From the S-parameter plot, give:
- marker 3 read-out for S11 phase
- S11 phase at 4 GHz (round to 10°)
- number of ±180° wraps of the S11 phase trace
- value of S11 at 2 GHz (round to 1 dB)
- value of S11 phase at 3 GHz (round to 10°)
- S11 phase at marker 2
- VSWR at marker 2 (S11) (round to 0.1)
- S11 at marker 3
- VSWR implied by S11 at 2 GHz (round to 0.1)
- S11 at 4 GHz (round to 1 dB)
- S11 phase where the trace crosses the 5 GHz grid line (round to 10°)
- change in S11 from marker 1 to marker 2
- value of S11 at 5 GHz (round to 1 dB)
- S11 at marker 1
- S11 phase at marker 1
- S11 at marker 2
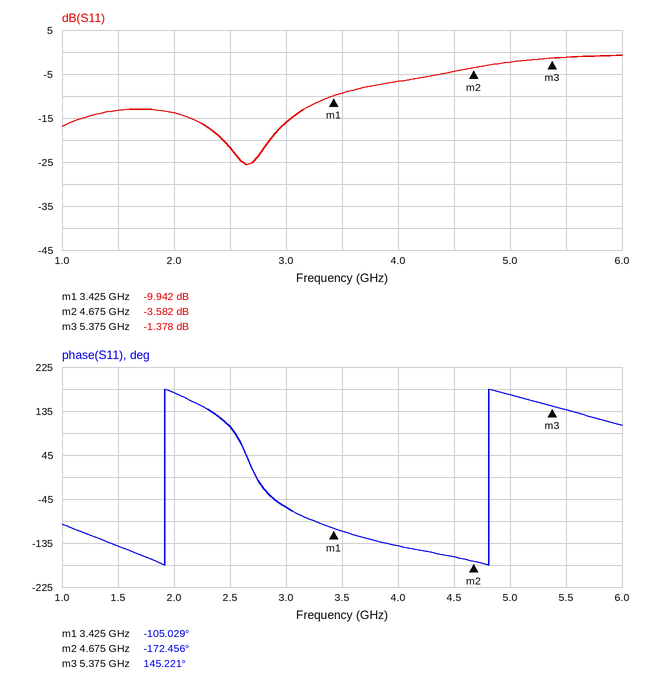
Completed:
145.221°
-140°
2
-14 dB
-60°
-172.456°
4.9
-1.378 dB
1.5
-7 dB
170°
6.360 dB
-2 dB
-9.942 dB
-105.029°
-3.582 dB
